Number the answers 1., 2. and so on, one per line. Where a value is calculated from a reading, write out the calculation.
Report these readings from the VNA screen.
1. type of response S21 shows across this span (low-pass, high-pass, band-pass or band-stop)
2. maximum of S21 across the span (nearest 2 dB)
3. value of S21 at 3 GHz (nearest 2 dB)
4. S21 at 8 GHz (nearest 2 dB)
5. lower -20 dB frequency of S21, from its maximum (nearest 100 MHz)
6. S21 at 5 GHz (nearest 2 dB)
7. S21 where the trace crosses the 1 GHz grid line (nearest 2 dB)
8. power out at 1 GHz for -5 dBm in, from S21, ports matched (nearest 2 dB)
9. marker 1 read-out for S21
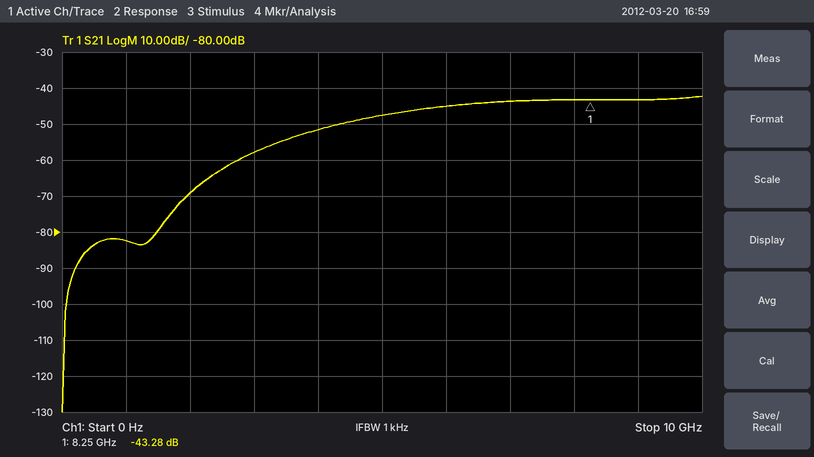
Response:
1. high-pass
2. -42 dB
3. -58 dB
4. -44 dB
5. 2.5 GHz
6. -48 dB
7. -82 dB
8. -5 dBm + (-82 dB) = -88 dBm
9. -43.28 dB
